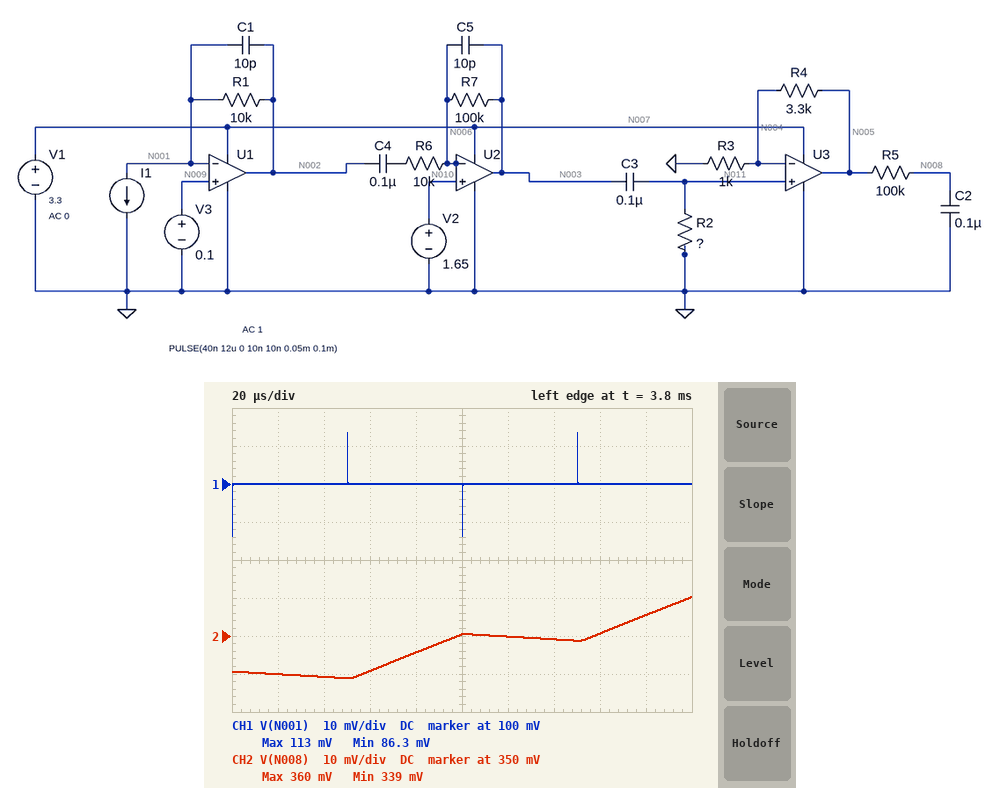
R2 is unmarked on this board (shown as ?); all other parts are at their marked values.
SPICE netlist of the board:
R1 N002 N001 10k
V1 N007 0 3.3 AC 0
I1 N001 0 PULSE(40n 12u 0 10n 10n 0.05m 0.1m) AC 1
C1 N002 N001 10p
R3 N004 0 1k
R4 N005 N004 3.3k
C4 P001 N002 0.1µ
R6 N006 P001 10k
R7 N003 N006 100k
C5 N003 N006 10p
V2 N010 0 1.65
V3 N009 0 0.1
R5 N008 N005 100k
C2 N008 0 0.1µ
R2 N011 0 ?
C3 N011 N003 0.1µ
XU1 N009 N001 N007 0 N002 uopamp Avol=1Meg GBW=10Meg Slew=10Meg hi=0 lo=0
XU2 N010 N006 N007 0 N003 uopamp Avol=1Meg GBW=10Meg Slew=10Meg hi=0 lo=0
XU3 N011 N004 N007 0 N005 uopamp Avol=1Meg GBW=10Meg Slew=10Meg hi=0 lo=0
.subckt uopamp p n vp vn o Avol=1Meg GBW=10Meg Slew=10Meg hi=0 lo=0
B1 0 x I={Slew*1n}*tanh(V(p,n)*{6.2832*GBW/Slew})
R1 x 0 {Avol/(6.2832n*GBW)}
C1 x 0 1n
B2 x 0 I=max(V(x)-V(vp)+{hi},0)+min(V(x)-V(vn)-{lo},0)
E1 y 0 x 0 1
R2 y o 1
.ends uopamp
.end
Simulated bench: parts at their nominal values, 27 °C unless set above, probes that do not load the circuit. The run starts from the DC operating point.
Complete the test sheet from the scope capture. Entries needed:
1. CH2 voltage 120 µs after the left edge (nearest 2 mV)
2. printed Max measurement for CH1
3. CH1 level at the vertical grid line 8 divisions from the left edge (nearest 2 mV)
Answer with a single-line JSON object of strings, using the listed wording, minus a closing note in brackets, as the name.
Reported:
{"CH2 voltage 120 µs after the left edge": "350 mV", "printed Max measurement for CH1": "113 mV", "CH1 level at the vertical grid line 8 divisions from the left edge": "100 mV"}
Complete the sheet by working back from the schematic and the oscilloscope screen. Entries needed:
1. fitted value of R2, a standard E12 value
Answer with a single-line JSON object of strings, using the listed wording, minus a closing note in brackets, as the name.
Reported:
{"fitted value of R2, a standard E12 value": "68 kΩ"}
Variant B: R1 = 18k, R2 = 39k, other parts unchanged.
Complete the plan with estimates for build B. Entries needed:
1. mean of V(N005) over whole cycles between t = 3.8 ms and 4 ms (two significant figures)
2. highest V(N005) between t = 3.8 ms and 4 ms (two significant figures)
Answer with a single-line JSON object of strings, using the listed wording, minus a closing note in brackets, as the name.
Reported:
{"mean of V(N005) over whole cycles between t = 3.8 ms and 4 ms": "1.6 V", "highest V(N005) between t = 3.8 ms and 4 ms": "3.3 V"}
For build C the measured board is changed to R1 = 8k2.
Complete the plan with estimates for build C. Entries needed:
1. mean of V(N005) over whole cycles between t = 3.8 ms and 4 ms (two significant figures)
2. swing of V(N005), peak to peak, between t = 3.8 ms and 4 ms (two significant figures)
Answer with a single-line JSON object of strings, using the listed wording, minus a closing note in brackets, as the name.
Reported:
{"mean of V(N005) over whole cycles between t = 3.8 ms and 4 ms": "1.1 V", "swing of V(N005), peak to peak, between t = 3.8 ms and 4 ms": "2.3 V"}
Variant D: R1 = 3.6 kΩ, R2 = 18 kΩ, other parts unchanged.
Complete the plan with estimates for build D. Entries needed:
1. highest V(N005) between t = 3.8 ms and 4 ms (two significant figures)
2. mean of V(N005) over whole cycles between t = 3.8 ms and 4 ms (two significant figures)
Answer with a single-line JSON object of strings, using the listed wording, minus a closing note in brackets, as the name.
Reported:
{"highest V(N005) between t = 3.8 ms and 4 ms": "1.0 V", "mean of V(N005) over whole cycles between t = 3.8 ms and 4 ms": "490 mV"}
